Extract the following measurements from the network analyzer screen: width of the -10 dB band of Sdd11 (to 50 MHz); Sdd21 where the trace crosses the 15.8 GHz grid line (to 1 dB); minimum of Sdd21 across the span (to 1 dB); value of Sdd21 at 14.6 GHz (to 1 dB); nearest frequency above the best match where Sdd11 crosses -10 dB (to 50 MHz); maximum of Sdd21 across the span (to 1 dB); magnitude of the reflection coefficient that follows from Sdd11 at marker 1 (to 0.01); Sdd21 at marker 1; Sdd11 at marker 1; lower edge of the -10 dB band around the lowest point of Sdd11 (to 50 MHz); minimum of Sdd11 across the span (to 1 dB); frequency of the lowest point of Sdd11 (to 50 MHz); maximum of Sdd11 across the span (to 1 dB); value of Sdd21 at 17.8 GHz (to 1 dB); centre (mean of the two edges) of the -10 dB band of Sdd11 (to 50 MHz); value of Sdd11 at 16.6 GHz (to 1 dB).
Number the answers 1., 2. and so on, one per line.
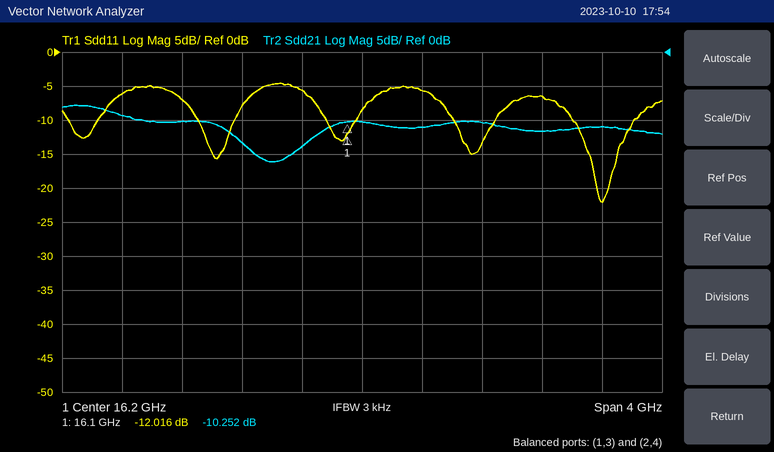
1. 400 MHz
2. -14 dB
3. -16 dB
4. -9 dB
5. 18.00 GHz
6. -8 dB
7. 0.25
8. -10.252 dB
9. -12.016 dB
10. 17.60 GHz
11. -22 dB
12. 17.80 GHz
13. -5 dB
14. -11 dB
15. 17.80 GHz
16. -6 dB
